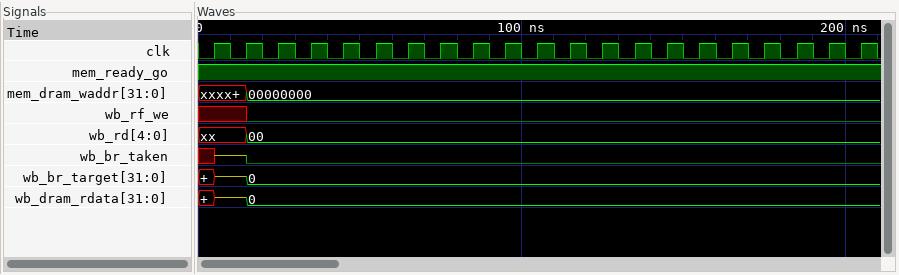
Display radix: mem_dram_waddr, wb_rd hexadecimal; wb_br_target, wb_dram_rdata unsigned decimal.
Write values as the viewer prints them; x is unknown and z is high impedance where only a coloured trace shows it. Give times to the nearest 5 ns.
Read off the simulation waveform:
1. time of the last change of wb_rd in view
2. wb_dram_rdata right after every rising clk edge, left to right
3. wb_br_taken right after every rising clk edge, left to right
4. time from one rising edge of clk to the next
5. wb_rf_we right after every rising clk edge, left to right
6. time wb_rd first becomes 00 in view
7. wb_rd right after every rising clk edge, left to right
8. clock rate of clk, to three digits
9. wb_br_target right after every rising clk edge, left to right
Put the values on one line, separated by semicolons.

15 ns; z, 0, 0, 0, 0, 0, 0, 0, 0, 0, 0, 0, 0, 0, 0, 0, 0, 0, 0, 0, 0; z 0 0 0 0 0 0 0 0 0 0 0 0 0 0 0 0 0 0 0 0; 10 ns; x 0 0 0 0 0 0 0 0 0 0 0 0 0 0 0 0 0 0 0 0; 15 ns; xx, 00, 00, 00, 00, 00, 00, 00, 00, 00, 00, 00, 00, 00, 00, 00, 00, 00, 00, 00, 00; 100 MHz; z, 0, 0, 0, 0, 0, 0, 0, 0, 0, 0, 0, 0, 0, 0, 0, 0, 0, 0, 0, 0
